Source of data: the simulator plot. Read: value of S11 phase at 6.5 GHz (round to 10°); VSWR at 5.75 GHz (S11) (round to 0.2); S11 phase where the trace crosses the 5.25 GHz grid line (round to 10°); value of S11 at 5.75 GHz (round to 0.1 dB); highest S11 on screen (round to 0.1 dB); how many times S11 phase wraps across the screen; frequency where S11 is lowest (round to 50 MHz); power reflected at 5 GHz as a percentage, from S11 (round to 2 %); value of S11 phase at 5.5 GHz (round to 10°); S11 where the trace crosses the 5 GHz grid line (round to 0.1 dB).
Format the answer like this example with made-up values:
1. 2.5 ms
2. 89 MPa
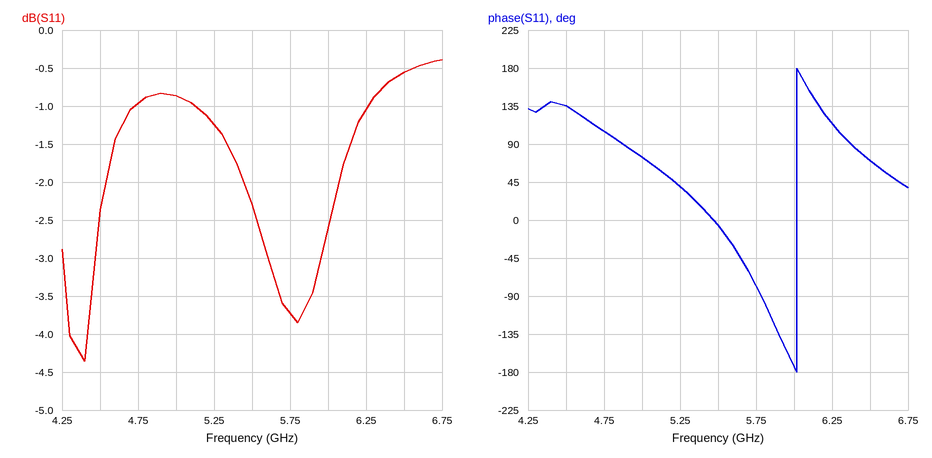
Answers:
1. 70°
2. 4.8
3. 40°
4. -3.7 dB
5. -0.4 dB
6. 1
7. 4.40 GHz
8. 82 %
9. -10°
10. -0.9 dB
